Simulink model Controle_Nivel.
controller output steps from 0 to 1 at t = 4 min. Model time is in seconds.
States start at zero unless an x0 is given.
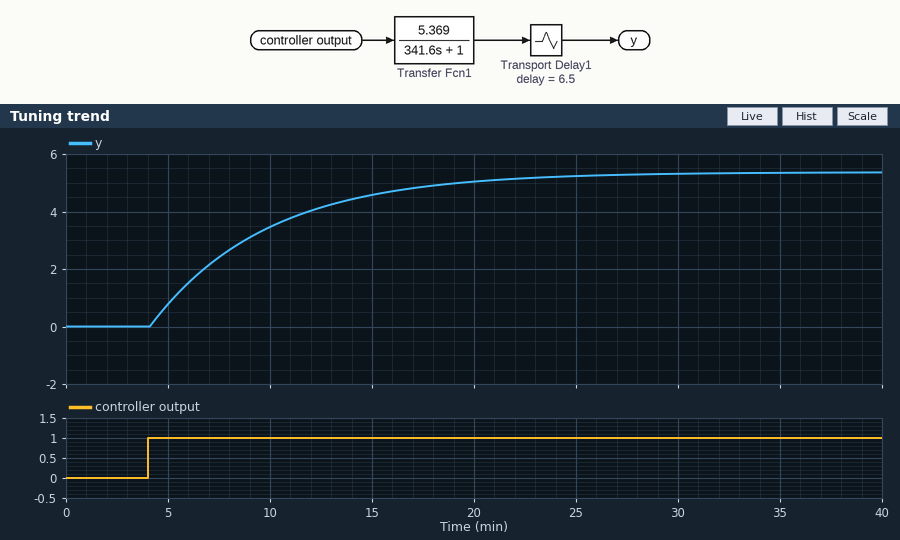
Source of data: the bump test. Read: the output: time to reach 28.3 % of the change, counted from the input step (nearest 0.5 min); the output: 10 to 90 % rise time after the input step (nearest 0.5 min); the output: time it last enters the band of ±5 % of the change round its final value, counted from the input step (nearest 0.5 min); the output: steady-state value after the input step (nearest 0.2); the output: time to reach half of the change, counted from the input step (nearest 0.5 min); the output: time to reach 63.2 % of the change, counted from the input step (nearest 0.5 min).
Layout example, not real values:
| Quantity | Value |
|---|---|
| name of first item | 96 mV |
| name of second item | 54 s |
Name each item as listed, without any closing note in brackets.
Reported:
| Quantity | Value |
|---|---|
| the output: time to reach 28.3 % of the change, counted from the input step | 2.0 min |
| the output: 10 to 90 % rise time after the input step | 12.5 min |
| the output: time it last enters the band of ±5 % of the change round its final value, counted from the input step | 17.0 min |
| the output: steady-state value after the input step | 5.4 |
| the output: time to reach half of the change, counted from the input step | 4.0 min |
| the output: time to reach 63.2 % of the change, counted from the input step | 6.0 min |
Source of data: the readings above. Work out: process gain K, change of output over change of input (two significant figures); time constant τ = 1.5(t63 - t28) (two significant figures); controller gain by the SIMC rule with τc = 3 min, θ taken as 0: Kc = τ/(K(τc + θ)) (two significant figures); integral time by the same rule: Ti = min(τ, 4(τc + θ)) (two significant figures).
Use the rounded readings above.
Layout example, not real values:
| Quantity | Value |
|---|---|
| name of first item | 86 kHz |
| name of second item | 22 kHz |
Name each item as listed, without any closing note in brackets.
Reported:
| Quantity | Value |
|---|---|
| process gain K, change of output over change of input | 5.4 |
| time constant τ = 1.5(t63 - t28) | 6.0 min |
| controller gain by the SIMC rule with τc = 3 min, θ taken as 0: Kc = τ/(K(τc + θ)) | 0.37 |
| integral time by the same rule: Ti = min(τ, 4(τc + θ)) | 6.0 min |
